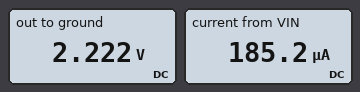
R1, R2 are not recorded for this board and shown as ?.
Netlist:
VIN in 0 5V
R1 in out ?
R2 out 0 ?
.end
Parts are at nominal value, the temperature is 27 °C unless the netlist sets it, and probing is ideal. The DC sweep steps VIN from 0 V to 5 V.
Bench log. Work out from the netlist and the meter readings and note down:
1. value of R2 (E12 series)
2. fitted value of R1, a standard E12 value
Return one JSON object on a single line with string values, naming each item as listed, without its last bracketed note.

{"value of R2": "12 kΩ", "fitted value of R1, a standard E12 value": "15 kΩ"}
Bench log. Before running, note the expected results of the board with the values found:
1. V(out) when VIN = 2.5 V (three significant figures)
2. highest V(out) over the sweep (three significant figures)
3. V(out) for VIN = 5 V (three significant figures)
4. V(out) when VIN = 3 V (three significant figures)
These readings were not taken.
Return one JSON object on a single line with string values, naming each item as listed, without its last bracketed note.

{"V(out) when VIN = 2.5 V": "1.11 V", "highest V(out) over the sweep": "2.22 V", "V(out) for VIN = 5 V": "2.22 V", "V(out) when VIN = 3 V": "1.33 V"}
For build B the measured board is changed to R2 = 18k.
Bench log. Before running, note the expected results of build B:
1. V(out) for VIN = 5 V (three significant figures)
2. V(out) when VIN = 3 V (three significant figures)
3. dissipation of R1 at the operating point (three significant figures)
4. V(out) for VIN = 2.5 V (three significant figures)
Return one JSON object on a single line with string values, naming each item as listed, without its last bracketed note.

{"V(out) for VIN = 5 V": "2.73 V", "V(out) when VIN = 3 V": "1.64 V", "dissipation of R1 at the operating point": "344 µW", "V(out) for VIN = 2.5 V": "1.36 V"}
